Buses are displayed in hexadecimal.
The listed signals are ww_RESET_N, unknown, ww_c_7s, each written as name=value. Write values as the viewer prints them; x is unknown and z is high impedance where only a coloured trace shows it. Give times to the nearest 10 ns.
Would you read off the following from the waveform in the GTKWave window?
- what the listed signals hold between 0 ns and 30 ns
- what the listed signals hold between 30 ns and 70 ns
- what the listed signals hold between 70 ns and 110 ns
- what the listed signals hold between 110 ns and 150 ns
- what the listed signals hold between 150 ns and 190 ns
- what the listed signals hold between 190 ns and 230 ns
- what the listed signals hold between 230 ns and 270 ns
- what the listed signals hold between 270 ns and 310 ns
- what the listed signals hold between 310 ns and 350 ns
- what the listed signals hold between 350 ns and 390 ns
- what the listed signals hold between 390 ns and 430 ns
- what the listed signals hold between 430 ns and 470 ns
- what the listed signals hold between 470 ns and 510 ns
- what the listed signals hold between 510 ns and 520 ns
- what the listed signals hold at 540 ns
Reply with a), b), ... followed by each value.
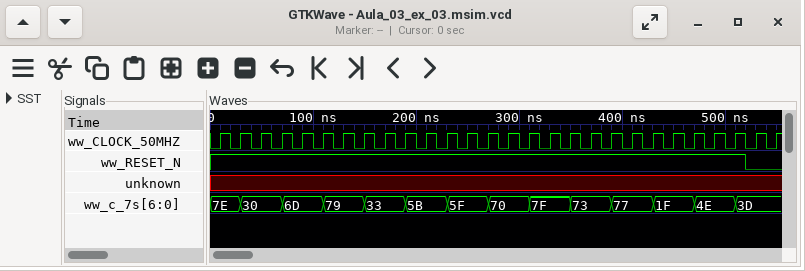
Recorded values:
a) ww_RESET_N=1, unknown=x, ww_c_7s=7E
b) ww_RESET_N=1, unknown=x, ww_c_7s=30
c) ww_RESET_N=1, unknown=x, ww_c_7s=6D
d) ww_RESET_N=1, unknown=x, ww_c_7s=79
e) ww_RESET_N=1, unknown=x, ww_c_7s=33
f) ww_RESET_N=1, unknown=x, ww_c_7s=5B
g) ww_RESET_N=1, unknown=x, ww_c_7s=5F
h) ww_RESET_N=1, unknown=x, ww_c_7s=70
i) ww_RESET_N=1, unknown=x, ww_c_7s=7F
j) ww_RESET_N=1, unknown=x, ww_c_7s=73
k) ww_RESET_N=1, unknown=x, ww_c_7s=77
l) ww_RESET_N=1, unknown=x, ww_c_7s=1F
m) ww_RESET_N=1, unknown=x, ww_c_7s=4E
n) ww_RESET_N=1, unknown=x, ww_c_7s=3D
o) ww_RESET_N=0, unknown=x, ww_c_7s=3D
